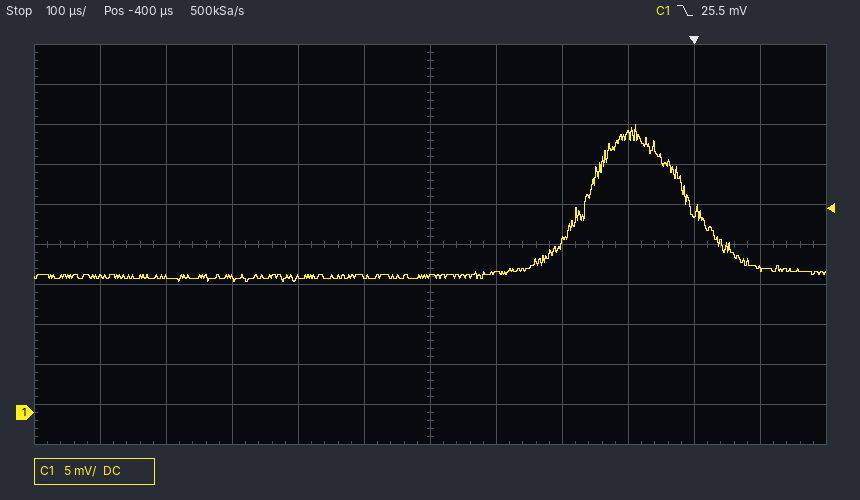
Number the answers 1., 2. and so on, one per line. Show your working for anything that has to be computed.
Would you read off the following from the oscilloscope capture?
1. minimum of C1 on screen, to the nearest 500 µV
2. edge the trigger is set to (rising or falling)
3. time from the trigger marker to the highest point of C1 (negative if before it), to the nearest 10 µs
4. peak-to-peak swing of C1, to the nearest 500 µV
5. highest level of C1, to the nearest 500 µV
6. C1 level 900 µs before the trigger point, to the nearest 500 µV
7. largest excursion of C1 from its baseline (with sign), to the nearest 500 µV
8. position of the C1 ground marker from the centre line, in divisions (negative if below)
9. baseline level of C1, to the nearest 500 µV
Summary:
1. 16.5 mV
2. falling
3. -90 µs
4. 36.0 mV − (16.5 mV) = 19.5 mV
5. 36.0 mV
6. 17.0 mV
7. 36.0 mV − (17.0 mV) = +19.0 mV
8. -4.2 div
9. 17.0 mV
